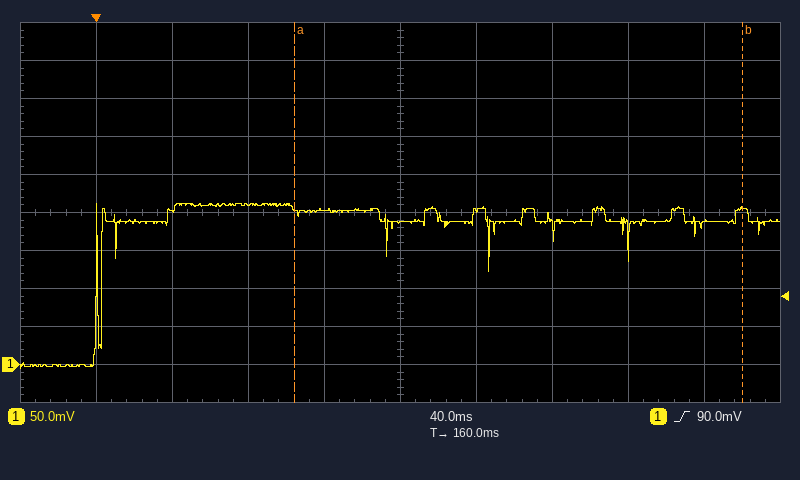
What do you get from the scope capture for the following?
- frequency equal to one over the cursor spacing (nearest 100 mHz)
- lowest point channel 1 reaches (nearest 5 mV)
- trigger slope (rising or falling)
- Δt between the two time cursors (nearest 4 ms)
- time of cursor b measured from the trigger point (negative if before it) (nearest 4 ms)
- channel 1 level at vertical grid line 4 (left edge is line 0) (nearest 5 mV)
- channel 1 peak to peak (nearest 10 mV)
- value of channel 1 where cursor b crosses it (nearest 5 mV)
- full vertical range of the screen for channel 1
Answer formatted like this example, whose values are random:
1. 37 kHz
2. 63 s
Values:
1. 4.2 Hz
2. -5 mV
3. rising
4. 236 ms
5. +340 ms
6. 205 mV
7. 220 mV
8. 205 mV
9. 500 mV
